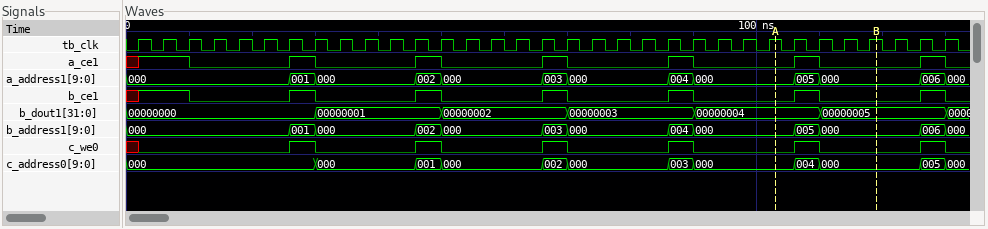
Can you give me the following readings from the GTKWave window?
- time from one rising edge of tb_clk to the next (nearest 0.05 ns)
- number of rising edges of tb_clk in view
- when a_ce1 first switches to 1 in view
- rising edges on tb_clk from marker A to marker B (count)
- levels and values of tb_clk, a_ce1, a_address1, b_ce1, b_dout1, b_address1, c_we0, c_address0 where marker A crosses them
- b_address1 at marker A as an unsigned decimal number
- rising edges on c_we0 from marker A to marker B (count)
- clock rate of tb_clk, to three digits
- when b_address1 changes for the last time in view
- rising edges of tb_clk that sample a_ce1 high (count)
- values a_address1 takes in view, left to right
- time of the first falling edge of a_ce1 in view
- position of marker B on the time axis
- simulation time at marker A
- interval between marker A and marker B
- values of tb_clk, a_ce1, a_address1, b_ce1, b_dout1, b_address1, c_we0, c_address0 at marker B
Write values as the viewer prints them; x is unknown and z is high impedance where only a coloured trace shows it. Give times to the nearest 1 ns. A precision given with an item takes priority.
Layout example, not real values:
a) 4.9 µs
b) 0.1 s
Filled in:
a) 4 ns
b) 33
c) 2 ns
d) 4
e) tb_clk=1, a_ce1=0, a_address1=000, b_ce1=0, b_dout1=00000004, b_address1=000, c_we0=0, c_address0=000
f) 0
g) 1
h) 250 MHz
i) 130 ns
j) 8
k) 000, 001, 000, 002, 000, 003, 000, 004, 000, 005, 000, 006, 000
l) 10 ns
m) 119 ns
n) 103 ns
o) 16 ns
p) tb_clk=1, a_ce1=0, a_address1=000, b_ce1=0, b_dout1=00000005, b_address1=000, c_we0=0, c_address0=000
